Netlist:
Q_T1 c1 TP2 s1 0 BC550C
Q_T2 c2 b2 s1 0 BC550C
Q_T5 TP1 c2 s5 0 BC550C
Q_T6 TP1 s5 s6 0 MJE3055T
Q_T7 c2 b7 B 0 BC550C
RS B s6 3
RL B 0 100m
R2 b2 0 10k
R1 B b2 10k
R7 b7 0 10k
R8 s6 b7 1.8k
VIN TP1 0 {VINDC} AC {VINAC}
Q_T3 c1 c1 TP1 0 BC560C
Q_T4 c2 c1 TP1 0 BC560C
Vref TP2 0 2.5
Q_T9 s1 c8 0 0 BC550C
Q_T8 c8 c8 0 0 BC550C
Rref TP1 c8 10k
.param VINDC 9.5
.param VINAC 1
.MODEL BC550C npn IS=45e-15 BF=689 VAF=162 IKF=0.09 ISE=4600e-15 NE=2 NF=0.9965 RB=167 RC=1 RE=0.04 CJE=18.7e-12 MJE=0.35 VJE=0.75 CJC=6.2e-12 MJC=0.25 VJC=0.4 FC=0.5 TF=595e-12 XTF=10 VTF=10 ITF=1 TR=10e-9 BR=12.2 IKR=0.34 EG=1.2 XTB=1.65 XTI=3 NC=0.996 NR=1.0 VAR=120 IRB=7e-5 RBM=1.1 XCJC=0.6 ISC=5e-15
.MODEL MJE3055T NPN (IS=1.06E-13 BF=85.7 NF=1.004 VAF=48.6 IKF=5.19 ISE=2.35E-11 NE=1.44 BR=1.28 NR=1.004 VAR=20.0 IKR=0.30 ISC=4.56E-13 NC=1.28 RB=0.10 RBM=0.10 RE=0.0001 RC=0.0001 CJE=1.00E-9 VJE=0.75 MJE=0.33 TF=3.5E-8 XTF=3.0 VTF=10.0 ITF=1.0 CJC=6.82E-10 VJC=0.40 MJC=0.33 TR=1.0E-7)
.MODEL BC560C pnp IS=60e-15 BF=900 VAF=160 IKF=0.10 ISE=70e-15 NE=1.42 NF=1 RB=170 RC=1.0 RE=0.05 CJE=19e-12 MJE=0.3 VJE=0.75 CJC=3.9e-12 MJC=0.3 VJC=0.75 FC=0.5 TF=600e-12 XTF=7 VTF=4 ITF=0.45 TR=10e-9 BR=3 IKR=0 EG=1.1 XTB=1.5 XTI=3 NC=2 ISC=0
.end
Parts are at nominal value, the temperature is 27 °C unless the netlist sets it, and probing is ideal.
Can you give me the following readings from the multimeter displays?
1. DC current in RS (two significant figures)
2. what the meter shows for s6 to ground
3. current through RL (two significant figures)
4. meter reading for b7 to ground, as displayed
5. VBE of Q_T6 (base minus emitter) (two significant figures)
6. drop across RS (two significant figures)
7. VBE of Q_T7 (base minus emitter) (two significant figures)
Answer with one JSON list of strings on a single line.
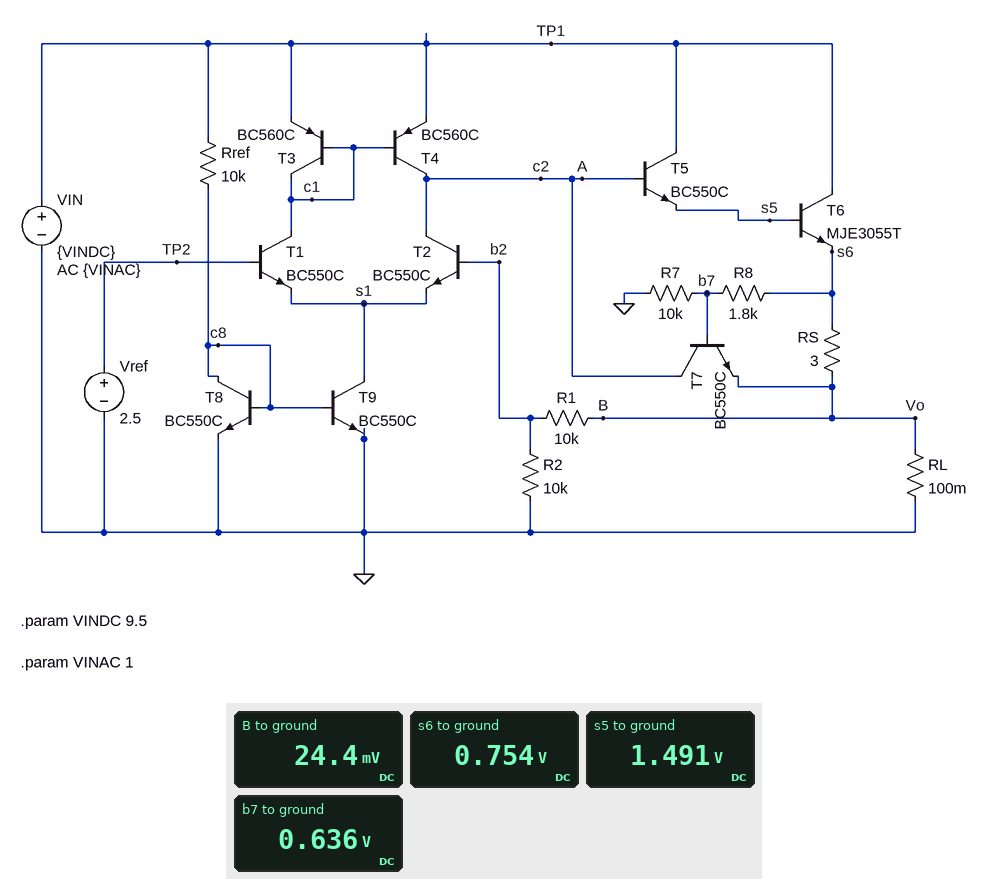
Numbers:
["240 mA", "0.754 V", "240 mA", "0.636 V", "740 mV", "730 mV", "610 mV"]
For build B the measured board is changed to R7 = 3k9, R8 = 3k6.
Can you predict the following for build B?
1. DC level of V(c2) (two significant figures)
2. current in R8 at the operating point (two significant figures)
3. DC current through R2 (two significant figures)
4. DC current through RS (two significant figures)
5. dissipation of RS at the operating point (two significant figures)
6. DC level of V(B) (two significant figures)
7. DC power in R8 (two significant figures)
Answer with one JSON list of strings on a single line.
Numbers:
["2.7 V", "170 µA", "2.0 µA", "410 mA", "500 mW", "41 mV", "100 µW"]
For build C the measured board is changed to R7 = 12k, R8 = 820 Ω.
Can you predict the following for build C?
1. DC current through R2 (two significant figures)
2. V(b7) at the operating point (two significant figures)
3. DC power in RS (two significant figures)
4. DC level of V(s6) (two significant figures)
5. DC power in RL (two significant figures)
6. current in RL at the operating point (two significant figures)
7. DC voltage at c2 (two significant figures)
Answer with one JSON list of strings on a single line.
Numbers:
["1.1 µA", "630 mV", "140 mW", "680 mV", "4.8 mW", "220 mA", "2.1 V"]
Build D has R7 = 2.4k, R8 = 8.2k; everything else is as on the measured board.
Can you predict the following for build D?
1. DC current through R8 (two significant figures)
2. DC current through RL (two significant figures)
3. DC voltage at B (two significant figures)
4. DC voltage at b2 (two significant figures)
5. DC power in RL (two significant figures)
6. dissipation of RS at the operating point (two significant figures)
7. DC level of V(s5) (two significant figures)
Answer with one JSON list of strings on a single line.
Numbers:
["300 µA", "1.0 A", "100 mV", "51 mV", "100 mW", "3.1 W", "3.9 V"]
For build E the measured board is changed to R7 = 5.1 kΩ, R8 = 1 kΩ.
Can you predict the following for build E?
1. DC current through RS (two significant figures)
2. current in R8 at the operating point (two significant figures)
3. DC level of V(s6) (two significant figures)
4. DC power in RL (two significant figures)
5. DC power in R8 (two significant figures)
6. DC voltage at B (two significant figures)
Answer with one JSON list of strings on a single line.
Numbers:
["250 mA", "130 µA", "760 mV", "6.1 mW", "16 µW", "25 mV"]
